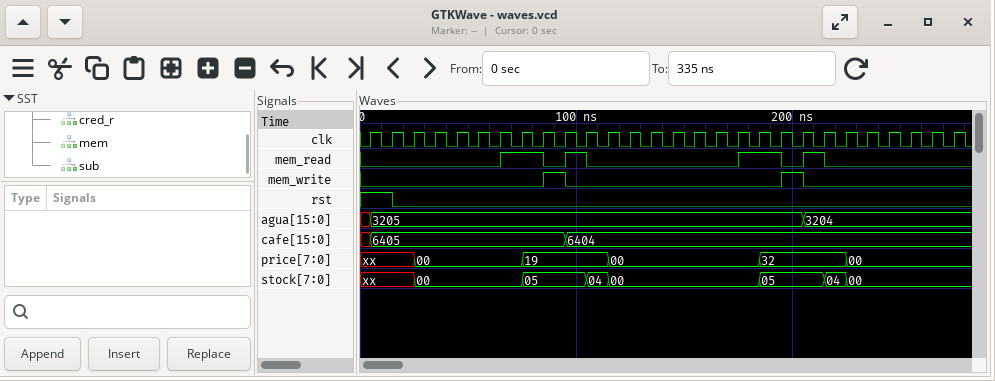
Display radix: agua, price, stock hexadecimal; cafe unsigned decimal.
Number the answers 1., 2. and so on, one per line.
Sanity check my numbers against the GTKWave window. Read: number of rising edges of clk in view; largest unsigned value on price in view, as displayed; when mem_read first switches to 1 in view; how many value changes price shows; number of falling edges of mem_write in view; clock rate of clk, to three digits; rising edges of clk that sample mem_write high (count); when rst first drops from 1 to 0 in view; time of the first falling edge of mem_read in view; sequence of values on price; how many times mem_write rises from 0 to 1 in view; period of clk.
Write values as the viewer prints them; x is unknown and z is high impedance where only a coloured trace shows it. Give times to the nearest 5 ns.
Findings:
1. 28
2. 32
3. 65 ns
4. 5
5. 2
6. 100 MHz
7. 2
8. 15 ns
9. 85 ns
10. xx, 00, 19, 00, 32, 00
11. 2
12. 10 ns
